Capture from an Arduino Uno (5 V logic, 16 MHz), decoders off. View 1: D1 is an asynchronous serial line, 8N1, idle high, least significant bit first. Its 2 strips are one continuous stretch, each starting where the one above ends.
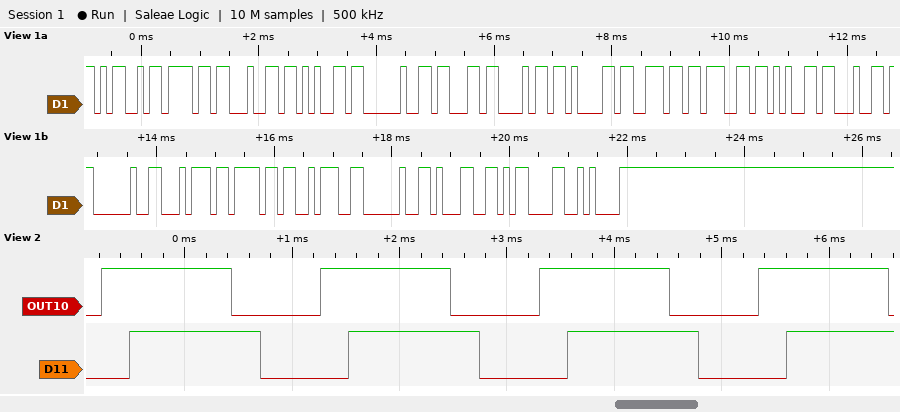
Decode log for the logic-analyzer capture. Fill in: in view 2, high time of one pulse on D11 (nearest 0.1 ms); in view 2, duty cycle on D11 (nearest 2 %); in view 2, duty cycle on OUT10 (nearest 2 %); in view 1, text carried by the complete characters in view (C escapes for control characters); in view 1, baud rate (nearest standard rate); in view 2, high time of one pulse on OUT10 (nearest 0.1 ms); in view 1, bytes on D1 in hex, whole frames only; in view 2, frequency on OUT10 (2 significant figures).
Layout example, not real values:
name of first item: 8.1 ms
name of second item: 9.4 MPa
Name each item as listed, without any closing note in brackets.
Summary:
in view 2, high time of one pulse on D11: 1.2 ms
in view 2, duty cycle on D11: 60 %
in view 2, duty cycle on OUT10: 60 %
in view 1, text carried by the complete characters in view: "Mode changed to: 1\r\n"
in view 1, baud rate: 9600 baud
in view 2, high time of one pulse on OUT10: 1.2 ms
in view 1, bytes on D1 in hex, whole frames only: 4D 6F 64 65 20 63 68 61 6E 67 65 64 20 74 6F 3A 20 31 0D 0A
in view 2, frequency on OUT10: 490 Hz
